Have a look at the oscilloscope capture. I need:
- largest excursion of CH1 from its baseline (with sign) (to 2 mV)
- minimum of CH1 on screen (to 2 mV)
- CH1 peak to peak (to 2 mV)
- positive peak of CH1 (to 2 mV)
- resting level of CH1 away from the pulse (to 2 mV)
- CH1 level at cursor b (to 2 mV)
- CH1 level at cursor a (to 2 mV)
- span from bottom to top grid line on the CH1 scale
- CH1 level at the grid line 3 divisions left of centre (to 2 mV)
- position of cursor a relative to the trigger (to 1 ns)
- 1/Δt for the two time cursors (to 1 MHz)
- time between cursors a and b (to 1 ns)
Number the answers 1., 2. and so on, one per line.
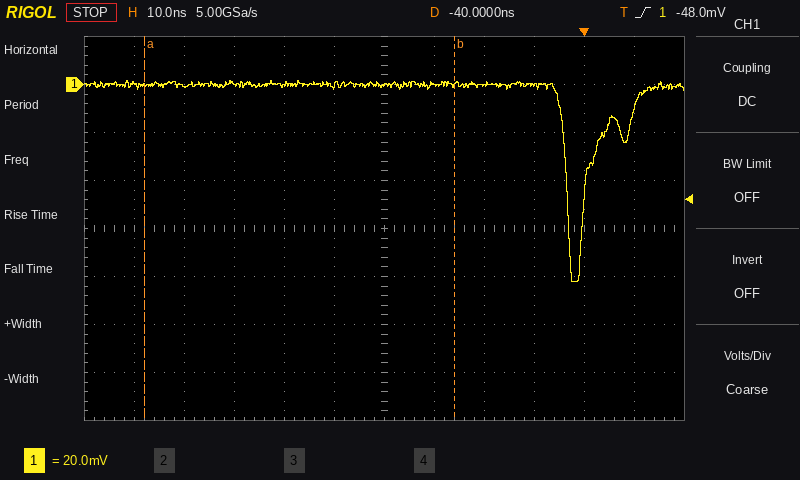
1. -82 mV
2. -82 mV
3. 84 mV
4. 2 mV
5. 0 mV
6. 0 mV
7. 0 mV
8. 160 mV
9. 0 mV
10. -88 ns
11. 16 MHz
12. 62 ns
